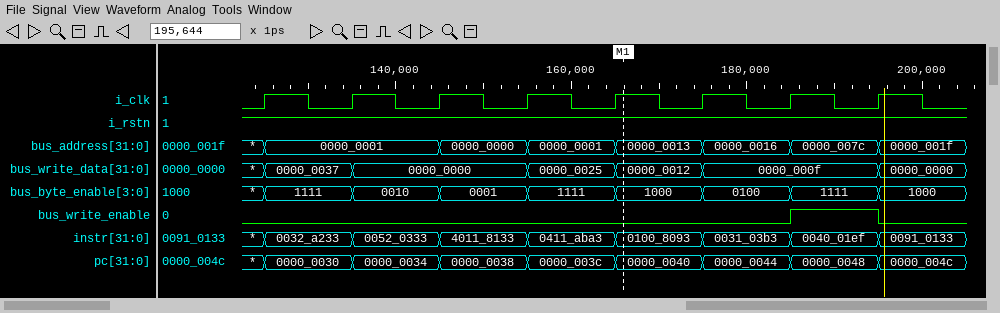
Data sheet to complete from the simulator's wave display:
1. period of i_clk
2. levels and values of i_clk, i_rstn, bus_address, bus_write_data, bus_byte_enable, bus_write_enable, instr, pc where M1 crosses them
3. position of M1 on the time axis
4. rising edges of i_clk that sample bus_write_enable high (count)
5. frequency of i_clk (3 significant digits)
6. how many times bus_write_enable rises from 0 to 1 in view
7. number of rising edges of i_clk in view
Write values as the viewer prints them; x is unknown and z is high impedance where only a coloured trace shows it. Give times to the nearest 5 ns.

10 ns
i_clk=1, i_rstn=1, bus_address=0000_0013, bus_write_data=0000_0012, bus_byte_enable=1000, bus_write_enable=0, instr=0100_8093, pc=0000_0040
165 ns
1
100 MHz
1
8
